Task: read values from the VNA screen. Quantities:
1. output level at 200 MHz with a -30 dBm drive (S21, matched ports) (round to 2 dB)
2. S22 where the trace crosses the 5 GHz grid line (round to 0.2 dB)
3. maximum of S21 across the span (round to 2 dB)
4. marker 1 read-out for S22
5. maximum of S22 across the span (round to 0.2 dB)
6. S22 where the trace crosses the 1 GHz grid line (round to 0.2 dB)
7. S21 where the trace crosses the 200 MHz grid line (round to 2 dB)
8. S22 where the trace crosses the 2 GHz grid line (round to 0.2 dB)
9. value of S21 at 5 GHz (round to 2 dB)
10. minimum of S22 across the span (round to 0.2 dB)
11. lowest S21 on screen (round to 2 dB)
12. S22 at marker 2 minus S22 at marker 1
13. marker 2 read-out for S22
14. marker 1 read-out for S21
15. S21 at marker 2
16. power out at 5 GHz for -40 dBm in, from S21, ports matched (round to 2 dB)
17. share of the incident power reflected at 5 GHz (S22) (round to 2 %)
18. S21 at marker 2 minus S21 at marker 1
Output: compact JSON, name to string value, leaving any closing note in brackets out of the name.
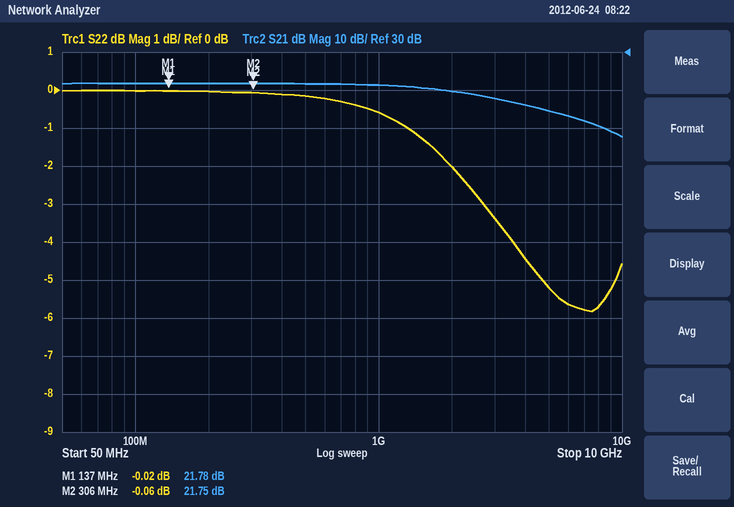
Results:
{"output level at 200 MHz with a -30 dBm drive (S21, matched ports)": "-8 dBm", "S22 where the trace crosses the 5 GHz grid line": "-5.2 dB", "maximum of S21 across the span": "22 dB", "marker 1 read-out for S22": "-0.02 dB", "maximum of S22 across the span": "0.0 dB", "S22 where the trace crosses the 1 GHz grid line": "-0.6 dB", "S21 where the trace crosses the 200 MHz grid line": "22 dB", "S22 where the trace crosses the 2 GHz grid line": "-2.0 dB", "value of S21 at 5 GHz": "14 dB", "minimum of S22 across the span": "-5.8 dB", "lowest S21 on screen": "8 dB", "S22 at marker 2 minus S22 at marker 1": "-0.04 dB", "marker 2 read-out for S22": "-0.06 dB", "marker 1 read-out for S21": "21.78 dB", "S21 at marker 2": "21.75 dB", "power out at 5 GHz for -40 dBm in, from S21, ports matched": "-26 dBm", "share of the incident power reflected at 5 GHz (S22)": "30 %", "S21 at marker 2 minus S21 at marker 1": "-0.03 dB"}
